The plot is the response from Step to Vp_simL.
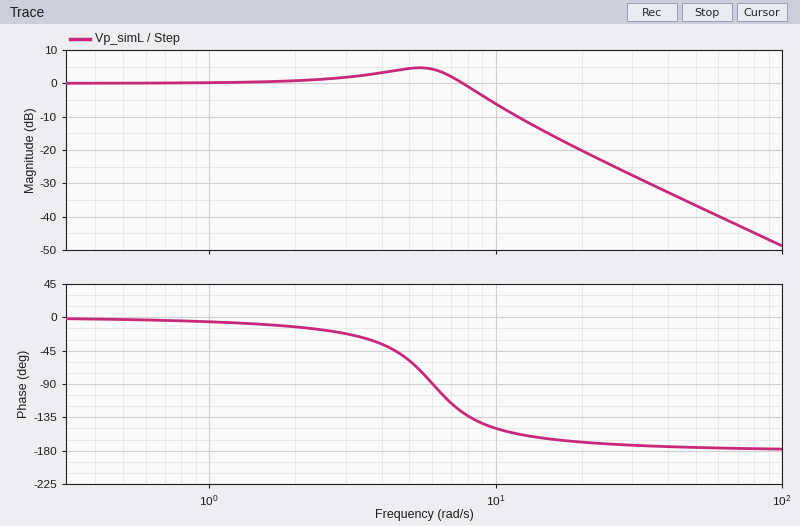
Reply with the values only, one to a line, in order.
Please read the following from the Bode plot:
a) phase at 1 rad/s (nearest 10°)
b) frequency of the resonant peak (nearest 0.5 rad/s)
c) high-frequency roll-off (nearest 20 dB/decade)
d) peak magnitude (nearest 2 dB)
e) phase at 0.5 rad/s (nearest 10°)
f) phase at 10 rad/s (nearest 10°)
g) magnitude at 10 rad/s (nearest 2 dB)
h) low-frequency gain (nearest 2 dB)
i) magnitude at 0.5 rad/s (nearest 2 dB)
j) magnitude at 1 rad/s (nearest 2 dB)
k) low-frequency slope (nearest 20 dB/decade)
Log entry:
-10°
5.5 rad/s
-40 dB/decade
4 dB
0°
-150°
-6 dB
0 dB
0 dB
0 dB
0 dB/decade
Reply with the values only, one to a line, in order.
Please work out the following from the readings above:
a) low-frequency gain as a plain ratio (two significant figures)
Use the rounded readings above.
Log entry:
1.0
